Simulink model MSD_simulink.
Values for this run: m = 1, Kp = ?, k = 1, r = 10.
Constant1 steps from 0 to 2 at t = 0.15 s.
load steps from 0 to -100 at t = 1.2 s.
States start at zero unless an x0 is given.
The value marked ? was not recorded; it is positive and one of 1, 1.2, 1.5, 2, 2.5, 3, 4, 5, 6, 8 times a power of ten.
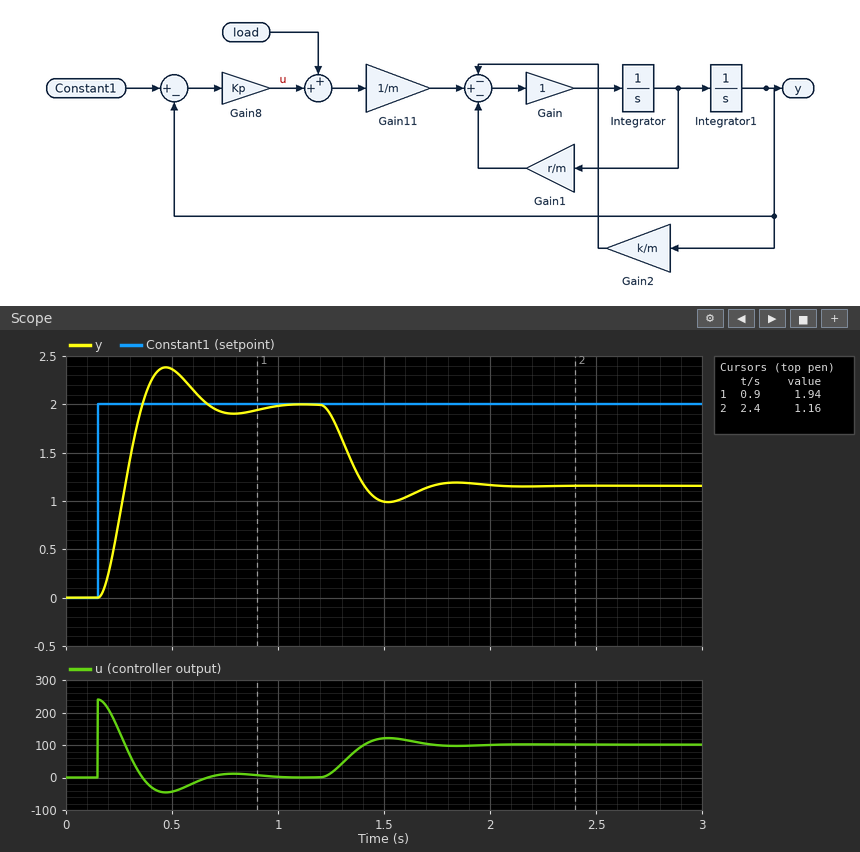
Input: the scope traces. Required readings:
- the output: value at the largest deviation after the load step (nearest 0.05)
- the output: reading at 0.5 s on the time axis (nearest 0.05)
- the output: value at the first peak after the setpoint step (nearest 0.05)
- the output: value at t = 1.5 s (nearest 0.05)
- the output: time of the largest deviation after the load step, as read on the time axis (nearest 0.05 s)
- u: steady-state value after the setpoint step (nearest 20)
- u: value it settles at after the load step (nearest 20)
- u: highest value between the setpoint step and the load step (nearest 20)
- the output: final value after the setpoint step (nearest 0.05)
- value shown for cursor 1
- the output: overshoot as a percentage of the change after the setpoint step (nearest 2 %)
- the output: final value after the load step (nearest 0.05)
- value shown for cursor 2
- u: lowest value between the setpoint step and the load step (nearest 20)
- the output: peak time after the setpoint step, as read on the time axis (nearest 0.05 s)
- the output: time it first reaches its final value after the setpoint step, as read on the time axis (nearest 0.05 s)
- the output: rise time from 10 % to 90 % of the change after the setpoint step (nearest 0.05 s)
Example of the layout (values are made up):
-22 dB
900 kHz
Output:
1.00
2.35
2.40
1.00
1.50 s
0
100
240
2.00
1.94
20 %
1.15
1.16
-40
0.45 s
0.35 s
0.15 s
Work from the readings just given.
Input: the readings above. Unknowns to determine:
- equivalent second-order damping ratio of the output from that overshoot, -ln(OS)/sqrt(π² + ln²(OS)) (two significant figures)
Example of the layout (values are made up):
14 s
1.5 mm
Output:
0.46
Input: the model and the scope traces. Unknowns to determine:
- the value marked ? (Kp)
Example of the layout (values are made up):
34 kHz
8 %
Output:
120
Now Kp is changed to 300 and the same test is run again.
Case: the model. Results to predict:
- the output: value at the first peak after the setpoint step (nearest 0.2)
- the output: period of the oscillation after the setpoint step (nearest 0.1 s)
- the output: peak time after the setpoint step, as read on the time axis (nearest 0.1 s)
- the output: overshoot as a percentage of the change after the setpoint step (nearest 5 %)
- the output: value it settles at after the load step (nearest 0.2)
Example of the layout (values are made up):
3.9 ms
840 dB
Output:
2.8
0.4 s
0.3 s
40 %
1.6
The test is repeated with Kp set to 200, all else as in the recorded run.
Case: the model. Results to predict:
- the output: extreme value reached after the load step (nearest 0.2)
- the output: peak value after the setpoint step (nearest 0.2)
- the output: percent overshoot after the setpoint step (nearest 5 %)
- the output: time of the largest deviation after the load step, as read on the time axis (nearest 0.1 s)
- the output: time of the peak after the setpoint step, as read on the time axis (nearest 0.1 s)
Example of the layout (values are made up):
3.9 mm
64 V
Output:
1.4
2.6
30 %
1.4 s
0.4 s
